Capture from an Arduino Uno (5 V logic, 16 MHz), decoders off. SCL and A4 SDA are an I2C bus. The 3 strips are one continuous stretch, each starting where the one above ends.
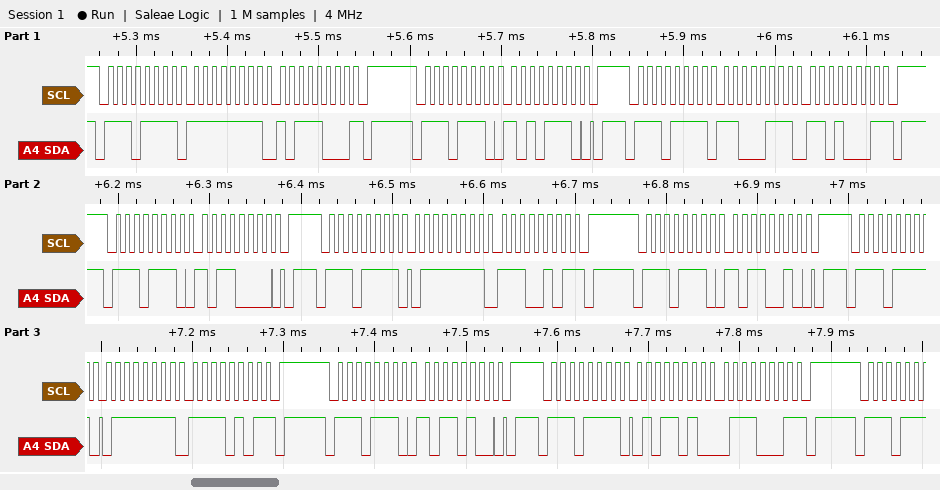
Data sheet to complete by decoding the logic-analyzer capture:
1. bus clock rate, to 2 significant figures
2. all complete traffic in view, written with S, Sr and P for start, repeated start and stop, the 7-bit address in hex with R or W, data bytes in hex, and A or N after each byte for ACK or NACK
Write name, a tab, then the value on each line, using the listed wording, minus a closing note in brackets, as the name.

bus clock rate, to 2 significant figures	100 kHz
all complete traffic in view, written with S, Sr and P for start, repeated start and stop, the 7-bit address in hex with R or W, data bytes in hex, and A or N after each byte for ACK or NACK	S 77R A FF A B8 N P S 77W A AE A P S 77R A C7 A D1 N P S 77W A B0 A P S 77R A 7F A E5 N P S 77W A B2 A P S 77R A 7F A F5 N P S 77W A B4 A P S 77R A 5A A 71 N P
